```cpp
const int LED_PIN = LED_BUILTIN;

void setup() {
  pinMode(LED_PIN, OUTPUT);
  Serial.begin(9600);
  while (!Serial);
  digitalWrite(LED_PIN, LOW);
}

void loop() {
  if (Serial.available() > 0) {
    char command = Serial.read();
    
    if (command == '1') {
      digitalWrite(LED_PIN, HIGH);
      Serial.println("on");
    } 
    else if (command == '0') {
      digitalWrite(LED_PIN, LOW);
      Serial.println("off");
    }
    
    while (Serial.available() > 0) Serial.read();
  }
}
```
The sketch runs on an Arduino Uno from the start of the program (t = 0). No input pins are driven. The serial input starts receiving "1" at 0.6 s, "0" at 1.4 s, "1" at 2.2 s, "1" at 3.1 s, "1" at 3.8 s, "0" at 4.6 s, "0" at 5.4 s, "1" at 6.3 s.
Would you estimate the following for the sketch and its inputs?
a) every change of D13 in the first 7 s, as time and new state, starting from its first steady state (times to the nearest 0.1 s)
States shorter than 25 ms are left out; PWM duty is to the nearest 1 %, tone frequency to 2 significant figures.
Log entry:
0 s low; 0.6 s high; 1.4 s low; 2.2 s high; 4.6 s low; 6.3 s high
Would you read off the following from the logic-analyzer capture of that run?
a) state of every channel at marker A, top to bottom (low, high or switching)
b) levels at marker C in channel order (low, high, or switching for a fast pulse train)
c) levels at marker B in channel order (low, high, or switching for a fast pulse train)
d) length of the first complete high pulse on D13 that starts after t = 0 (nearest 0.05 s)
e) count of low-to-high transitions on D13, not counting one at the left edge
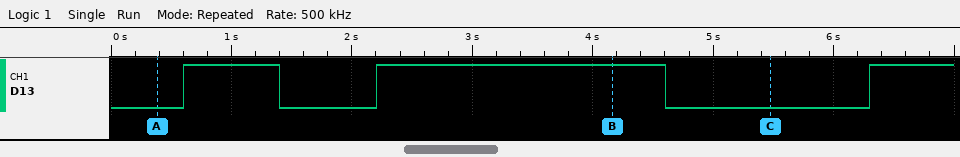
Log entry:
D13 low
D13 low
D13 high
0.80 s
3
